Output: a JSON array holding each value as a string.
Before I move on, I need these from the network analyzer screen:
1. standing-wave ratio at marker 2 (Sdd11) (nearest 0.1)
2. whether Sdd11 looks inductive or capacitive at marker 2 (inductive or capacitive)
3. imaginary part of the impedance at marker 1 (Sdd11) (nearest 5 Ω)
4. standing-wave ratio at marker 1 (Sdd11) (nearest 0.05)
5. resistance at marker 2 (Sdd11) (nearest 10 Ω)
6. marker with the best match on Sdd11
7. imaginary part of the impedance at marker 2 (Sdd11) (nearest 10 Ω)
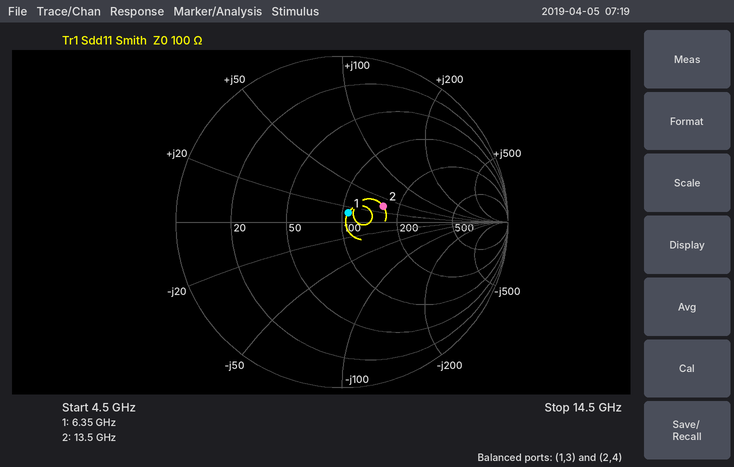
["1.7", "inductive", "+10 Ω", "1.15", "160 Ω", "marker 1", "+30 Ω"]
